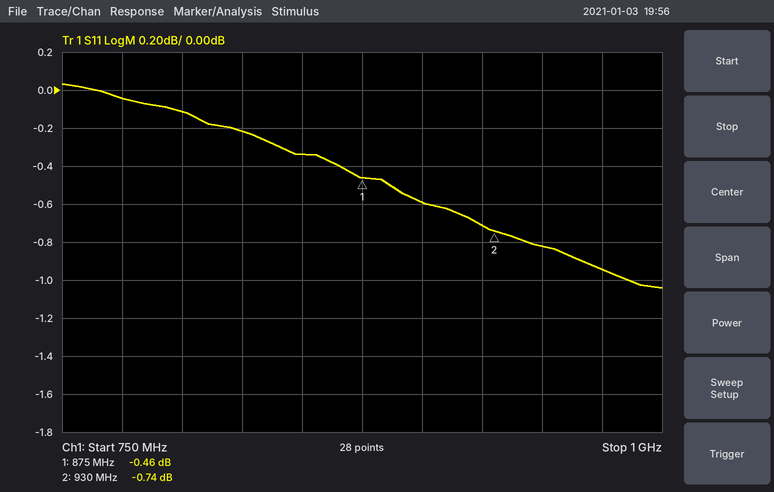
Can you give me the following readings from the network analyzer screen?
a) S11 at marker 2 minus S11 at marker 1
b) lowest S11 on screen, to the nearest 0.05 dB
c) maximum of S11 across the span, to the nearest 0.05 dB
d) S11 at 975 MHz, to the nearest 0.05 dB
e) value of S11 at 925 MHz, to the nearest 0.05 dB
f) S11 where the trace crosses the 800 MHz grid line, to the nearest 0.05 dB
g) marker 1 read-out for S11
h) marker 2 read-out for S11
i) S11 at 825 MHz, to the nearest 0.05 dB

-0.28 dB
-1.05 dB
0.05 dB
-0.95 dB
-0.70 dB
-0.10 dB
-0.46 dB
-0.74 dB
-0.20 dB
